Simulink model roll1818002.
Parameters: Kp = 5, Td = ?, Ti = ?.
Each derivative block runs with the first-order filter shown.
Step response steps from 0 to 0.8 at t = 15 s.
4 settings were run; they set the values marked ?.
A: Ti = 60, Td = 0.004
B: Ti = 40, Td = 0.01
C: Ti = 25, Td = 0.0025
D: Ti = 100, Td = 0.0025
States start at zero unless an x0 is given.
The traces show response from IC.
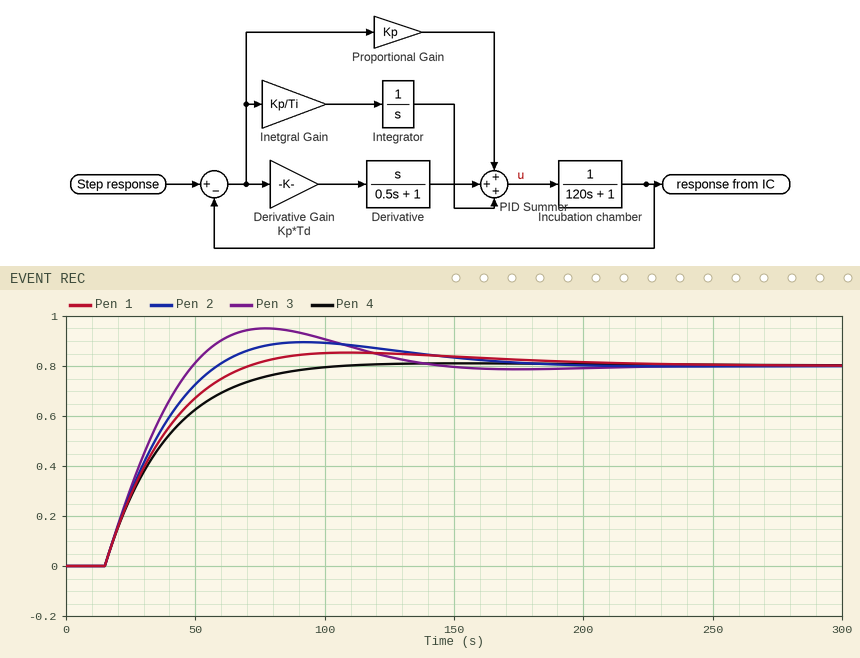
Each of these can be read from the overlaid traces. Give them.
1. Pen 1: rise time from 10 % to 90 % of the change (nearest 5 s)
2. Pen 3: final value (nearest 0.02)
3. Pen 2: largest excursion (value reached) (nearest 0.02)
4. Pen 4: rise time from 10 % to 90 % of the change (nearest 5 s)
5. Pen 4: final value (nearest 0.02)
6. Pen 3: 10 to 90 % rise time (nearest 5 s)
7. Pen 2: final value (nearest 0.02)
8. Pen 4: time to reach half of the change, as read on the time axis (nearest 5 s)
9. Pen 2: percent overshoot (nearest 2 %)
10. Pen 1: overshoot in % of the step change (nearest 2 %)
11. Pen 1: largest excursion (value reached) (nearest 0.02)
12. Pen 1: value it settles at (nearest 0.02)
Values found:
40 s
0.80
0.90
50 s
0.80
25 s
0.80
30 s
12 %
6 %
0.86
0.80
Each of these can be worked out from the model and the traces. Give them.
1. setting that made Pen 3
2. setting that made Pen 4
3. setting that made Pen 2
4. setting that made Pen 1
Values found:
C
D
B
A
